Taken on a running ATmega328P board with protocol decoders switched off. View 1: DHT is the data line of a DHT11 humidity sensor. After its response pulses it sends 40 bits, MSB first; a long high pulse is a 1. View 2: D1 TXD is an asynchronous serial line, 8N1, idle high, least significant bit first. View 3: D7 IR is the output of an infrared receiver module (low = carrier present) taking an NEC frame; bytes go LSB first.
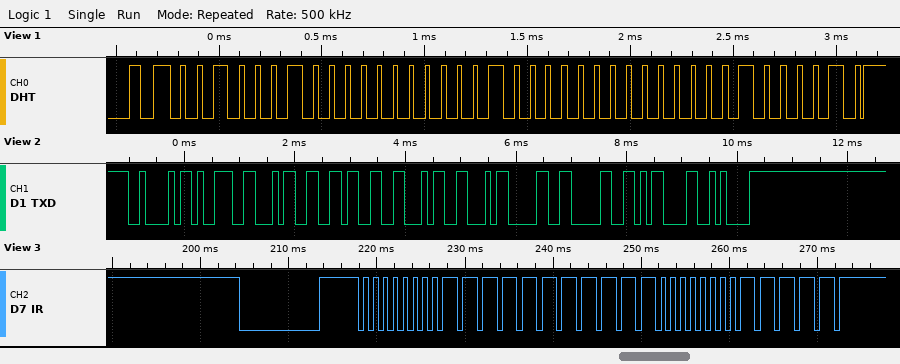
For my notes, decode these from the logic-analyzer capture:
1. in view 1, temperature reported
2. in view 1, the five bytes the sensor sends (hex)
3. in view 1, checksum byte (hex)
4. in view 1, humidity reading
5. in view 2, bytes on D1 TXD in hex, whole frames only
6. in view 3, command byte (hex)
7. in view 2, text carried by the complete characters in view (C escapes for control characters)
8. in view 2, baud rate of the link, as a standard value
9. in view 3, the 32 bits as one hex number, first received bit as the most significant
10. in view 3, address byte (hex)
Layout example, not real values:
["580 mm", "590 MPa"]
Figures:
["32.0 °C", "22 00 20 00 42", "0x42", "34 %", "0x42 0x39 0x34 0x36 0x46 0x46 0x30 0x30 0x0D 0x0A", "0x07", "\"B946FF00\\r\\n\"", "9600 baud", "0x00FFE01F", "0x00"]
